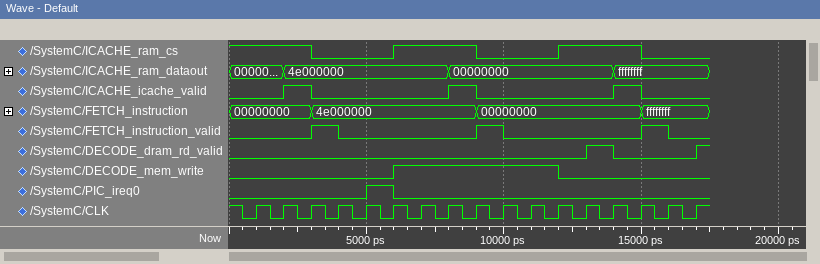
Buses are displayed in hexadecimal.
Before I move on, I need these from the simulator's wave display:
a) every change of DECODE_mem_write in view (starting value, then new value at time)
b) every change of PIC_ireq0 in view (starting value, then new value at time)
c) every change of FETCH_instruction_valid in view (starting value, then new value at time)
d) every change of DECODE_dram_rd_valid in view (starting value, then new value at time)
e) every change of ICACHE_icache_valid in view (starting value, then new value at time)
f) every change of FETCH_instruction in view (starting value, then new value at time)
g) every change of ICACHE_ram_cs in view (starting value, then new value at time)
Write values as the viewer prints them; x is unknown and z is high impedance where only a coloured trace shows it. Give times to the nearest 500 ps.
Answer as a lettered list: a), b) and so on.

a) 0, 1 at 6000 ps, 0 at 12000 ps
b) 0, 1 at 5000 ps, 0 at 6000 ps
c) 0, 1 at 3000 ps, 0 at 4000 ps, 1 at 9000 ps, 0 at 10000 ps, 1 at 15000 ps, 0 at 16000 ps
d) 0, 1 at 13000 ps, 0 at 14000 ps, 1 at 17000 ps
e) 0, 1 at 2000 ps, 0 at 3000 ps, 1 at 8000 ps, 0 at 9000 ps, 1 at 14000 ps, 0 at 15000 ps
f) 00000000, 4e000000 at 3000 ps, 00000000 at 9000 ps, ffffffff at 15000 ps
g) 1, 0 at 3000 ps, 1 at 6000 ps, 0 at 9000 ps, 1 at 12000 ps, 0 at 15000 ps
